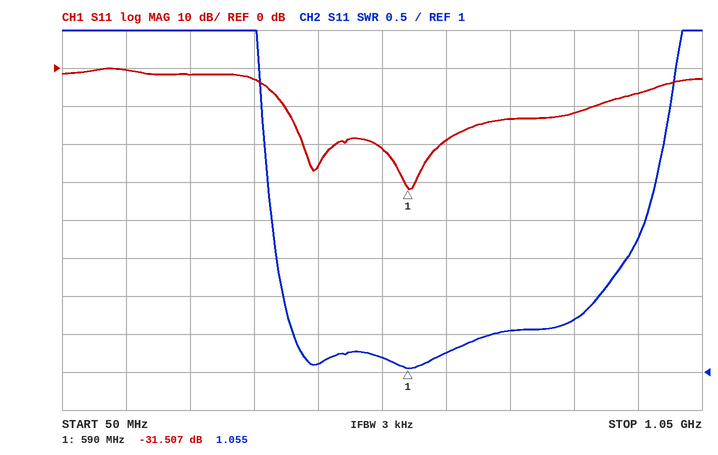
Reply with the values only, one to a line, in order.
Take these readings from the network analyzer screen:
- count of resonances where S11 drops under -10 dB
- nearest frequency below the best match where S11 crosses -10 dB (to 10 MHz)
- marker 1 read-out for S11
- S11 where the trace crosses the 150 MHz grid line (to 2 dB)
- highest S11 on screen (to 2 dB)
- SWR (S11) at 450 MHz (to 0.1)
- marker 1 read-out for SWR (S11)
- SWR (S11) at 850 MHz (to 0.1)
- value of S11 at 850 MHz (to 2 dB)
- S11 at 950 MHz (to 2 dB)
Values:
2
400 MHz
-31.507 dB
0 dB
0 dB
1.1
1.055
1.7
-12 dB
-6 dB
